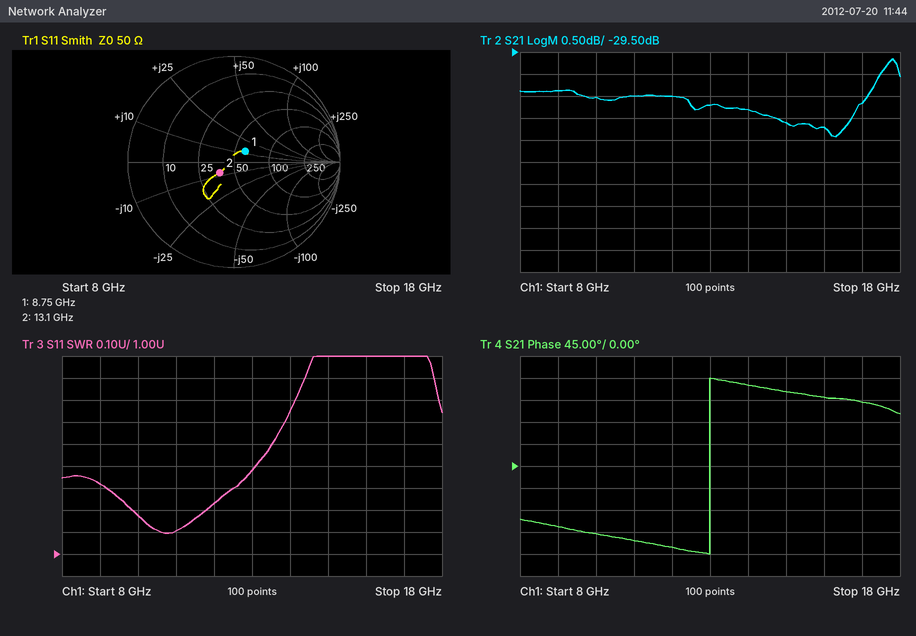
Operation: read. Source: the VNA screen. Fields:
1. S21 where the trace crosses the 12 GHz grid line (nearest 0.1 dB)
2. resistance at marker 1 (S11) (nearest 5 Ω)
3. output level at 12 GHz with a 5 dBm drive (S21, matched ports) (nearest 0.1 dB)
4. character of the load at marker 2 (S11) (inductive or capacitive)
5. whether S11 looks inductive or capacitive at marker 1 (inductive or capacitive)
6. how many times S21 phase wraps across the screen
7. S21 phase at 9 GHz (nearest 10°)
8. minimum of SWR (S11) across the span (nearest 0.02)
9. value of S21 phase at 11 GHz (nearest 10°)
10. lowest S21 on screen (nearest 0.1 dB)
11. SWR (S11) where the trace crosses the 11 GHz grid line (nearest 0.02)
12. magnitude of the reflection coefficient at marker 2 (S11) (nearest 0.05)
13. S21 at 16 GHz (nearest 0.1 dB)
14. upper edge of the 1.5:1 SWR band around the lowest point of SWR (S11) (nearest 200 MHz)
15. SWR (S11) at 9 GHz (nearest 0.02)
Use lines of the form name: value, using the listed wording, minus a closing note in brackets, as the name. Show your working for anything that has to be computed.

S21 where the trace crosses the 12 GHz grid line: -30.5 dB
resistance at marker 1 (S11): 60 Ω
output level at 12 GHz with a 5 dBm drive (S21, matched ports): 5 dBm + (-30.5 dB) = -25.5 dBm
character of the load at marker 2 (S11): capacitive
whether S11 looks inductive or capacitive at marker 1: inductive
how many times S21 phase wraps across the screen: 1
S21 phase at 9 GHz: -120°
minimum of SWR (S11) across the span: 1.10
value of S21 phase at 11 GHz: -150°
lowest S21 on screen: -31.4 dB
SWR (S11) where the trace crosses the 11 GHz grid line: 1.10
magnitude of the reflection coefficient at marker 2 (S11): 0.15
S21 at 16 GHz: -31.2 dB
upper edge of the 1.5:1 SWR band around the lowest point of SWR (S11): 13.6 GHz
SWR (S11) at 9 GHz: 1.32
